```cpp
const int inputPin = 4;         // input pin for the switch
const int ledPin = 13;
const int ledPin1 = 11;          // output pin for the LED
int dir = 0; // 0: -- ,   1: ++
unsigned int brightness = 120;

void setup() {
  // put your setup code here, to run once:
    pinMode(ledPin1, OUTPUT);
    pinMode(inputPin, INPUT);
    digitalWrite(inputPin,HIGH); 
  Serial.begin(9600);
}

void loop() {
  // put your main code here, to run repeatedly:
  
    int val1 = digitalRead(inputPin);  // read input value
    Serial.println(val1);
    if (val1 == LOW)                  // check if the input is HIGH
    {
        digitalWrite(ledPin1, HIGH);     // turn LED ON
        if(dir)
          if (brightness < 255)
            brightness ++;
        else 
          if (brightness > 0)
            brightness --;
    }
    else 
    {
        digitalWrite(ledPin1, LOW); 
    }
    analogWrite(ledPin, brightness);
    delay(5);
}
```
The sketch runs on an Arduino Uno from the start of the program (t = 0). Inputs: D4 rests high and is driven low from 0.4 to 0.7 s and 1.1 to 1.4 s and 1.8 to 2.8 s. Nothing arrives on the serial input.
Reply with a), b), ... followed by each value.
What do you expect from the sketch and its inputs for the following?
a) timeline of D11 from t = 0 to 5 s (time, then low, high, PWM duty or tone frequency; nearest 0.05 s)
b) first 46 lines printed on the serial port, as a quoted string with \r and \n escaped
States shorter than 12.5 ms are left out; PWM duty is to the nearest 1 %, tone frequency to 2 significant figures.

a) 0 s low; 0.4 s high; 0.7 s low; 1.1 s high; 1.4 s low; 1.8 s high; 2.8 s low
b) "1\r\n1\r\n1\r\n1\r\n1\r\n1\r\n1\r\n1\r\n1\r\n1\r\n1\r\n1\r\n1\r\n1\r\n1\r\n1\r\n1\r\n1\r\n1\r\n1\r\n1\r\n1\r\n1\r\n1\r\n1\r\n1\r\n1\r\n1\r\n1\r\n1\r\n1\r\n1\r\n1\r\n1\r\n1\r\n1\r\n1\r\n1\r\n1\r\n1\r\n1\r\n1\r\n1\r\n1\r\n1\r\n1\r\n"
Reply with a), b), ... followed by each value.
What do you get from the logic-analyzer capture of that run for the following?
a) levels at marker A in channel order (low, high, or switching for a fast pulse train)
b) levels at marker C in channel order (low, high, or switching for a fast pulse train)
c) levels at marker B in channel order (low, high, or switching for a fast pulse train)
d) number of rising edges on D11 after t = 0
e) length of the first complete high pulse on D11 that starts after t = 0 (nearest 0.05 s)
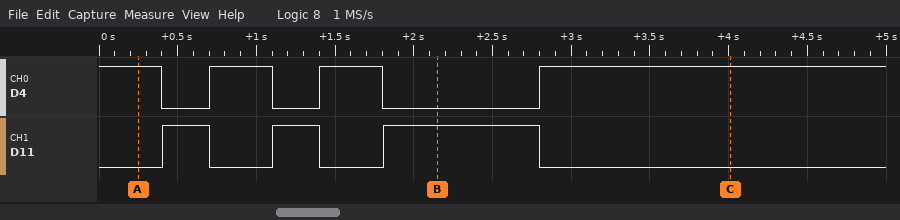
a) D4 high, D11 low
b) D4 high, D11 low
c) D4 low, D11 high
d) 3
e) 0.30 s
